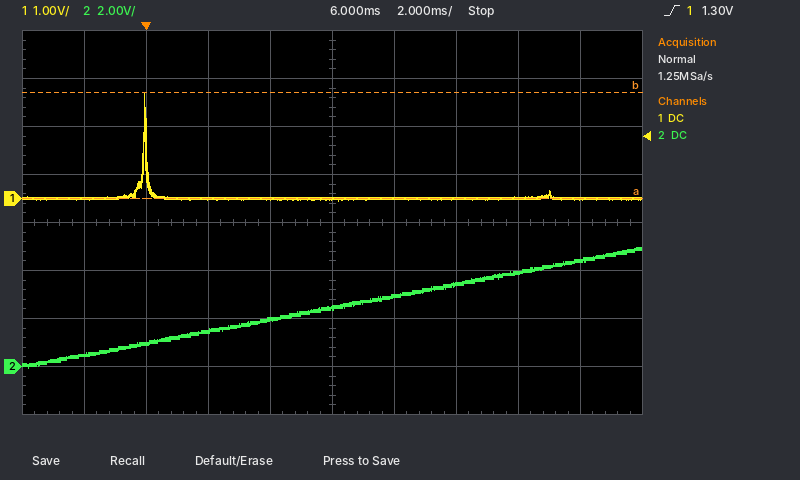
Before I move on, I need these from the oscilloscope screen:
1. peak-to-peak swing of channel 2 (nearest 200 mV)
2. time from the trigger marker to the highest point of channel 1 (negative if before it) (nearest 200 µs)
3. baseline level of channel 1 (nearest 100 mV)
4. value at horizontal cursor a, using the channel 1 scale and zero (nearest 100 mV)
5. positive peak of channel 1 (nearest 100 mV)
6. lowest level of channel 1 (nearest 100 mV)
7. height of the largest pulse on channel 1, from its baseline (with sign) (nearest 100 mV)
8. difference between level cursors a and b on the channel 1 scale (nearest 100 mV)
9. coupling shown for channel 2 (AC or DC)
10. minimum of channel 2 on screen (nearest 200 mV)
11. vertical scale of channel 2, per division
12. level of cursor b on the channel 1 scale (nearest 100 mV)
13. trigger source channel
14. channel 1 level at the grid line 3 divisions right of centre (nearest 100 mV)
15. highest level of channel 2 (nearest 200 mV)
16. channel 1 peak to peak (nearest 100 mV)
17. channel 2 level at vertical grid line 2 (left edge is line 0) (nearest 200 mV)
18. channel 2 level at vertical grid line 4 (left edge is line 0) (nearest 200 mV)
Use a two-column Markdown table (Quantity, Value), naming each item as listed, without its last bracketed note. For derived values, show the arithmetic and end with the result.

| Quantity | Value |
|---|---|
| peak-to-peak swing of channel 2 | 5.0 V − (0.0 V) = 5.0 V |
| time from the trigger marker to the highest point of channel 1 (negative if before it) | 0.0 ms |
| baseline level of channel 1 | 0.0 V |
| value at horizontal cursor a, using the channel 1 scale and zero | 0.0 V |
| positive peak of channel 1 | 2.2 V |
| lowest level of channel 1 | 0.0 V |
| height of the largest pulse on channel 1, from its baseline (with sign) | 2.2 V − (0.0 V) = +2.2 V |
| difference between level cursors a and b on the channel 1 scale | 2.2 V |
| coupling shown for channel 2 | DC |
| minimum of channel 2 on screen | 0.0 V |
| vertical scale of channel 2, per division | 2 V |
| level of cursor b on the channel 1 scale | 2.2 V |
| trigger source channel | channel 1 |
| channel 1 level at the grid line 3 divisions right of centre | 0.0 V |
| highest level of channel 2 | 5.0 V |
| channel 1 peak to peak | 2.2 V − (0.0 V) = 2.2 V |
| channel 2 level at vertical grid line 2 (left edge is line 0) | 1.0 V |
| channel 2 level at vertical grid line 4 (left edge is line 0) | 2.0 V |
